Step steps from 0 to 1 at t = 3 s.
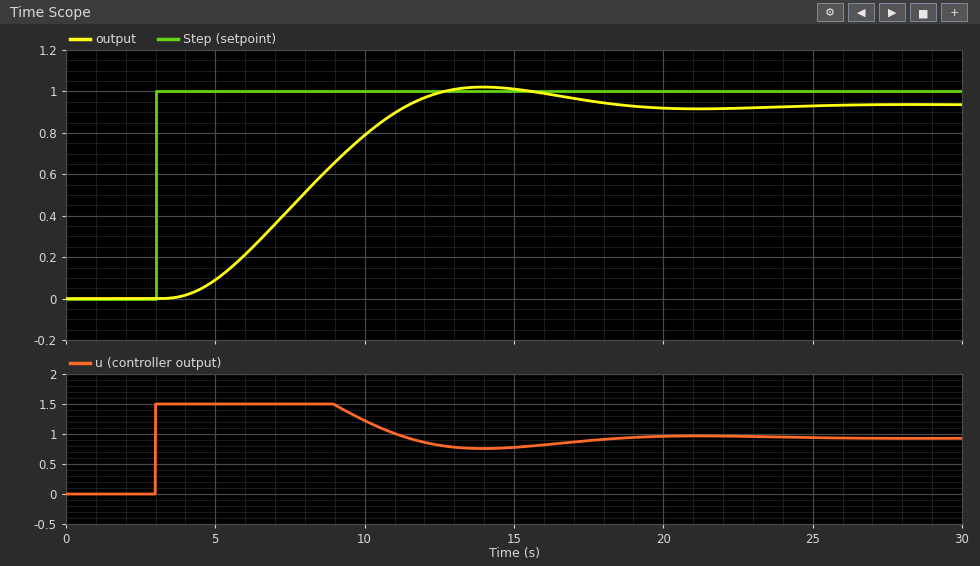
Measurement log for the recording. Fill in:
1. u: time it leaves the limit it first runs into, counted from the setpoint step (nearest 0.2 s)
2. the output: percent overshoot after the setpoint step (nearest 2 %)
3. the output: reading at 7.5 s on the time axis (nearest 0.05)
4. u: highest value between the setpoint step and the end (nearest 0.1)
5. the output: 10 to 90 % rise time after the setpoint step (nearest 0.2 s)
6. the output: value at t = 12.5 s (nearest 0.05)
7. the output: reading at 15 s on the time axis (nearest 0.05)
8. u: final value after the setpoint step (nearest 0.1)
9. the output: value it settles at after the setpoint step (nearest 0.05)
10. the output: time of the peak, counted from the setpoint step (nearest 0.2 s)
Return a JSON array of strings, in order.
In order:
["6.0 s", "10 %", "0.45", "1.5", "5.4 s", "1.00", "1.00", "0.9", "0.95", "11.0 s"]
